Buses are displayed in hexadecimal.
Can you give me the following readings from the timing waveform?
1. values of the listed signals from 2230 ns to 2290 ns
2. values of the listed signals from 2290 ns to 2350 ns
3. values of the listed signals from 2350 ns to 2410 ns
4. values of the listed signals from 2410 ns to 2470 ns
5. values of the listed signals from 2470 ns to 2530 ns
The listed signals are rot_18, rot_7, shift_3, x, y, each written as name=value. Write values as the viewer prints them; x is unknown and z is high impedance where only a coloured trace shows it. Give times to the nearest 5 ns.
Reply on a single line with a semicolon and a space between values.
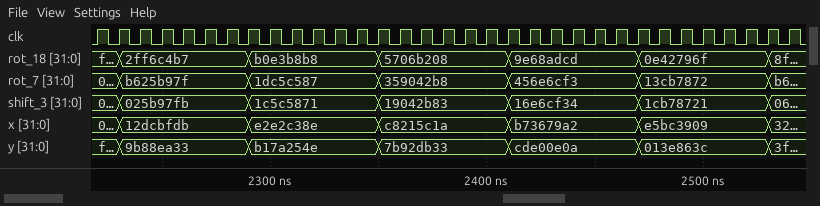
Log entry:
rot_18=2ff6c4b7, rot_7=b625b97f, shift_3=025b97fb, x=12dcbfdb, y=9b88ea33; rot_18=b0e3b8b8, rot_7=1dc5c587, shift_3=1c5c5871, x=e2e2c38e, y=b17a254e; rot_18=5706b208, rot_7=359042b8, shift_3=19042b83, x=c8215c1a, y=7b92db33; rot_18=9e68adcd, rot_7=456e6cf3, shift_3=16e6cf34, x=b73679a2, y=cde00e0a; rot_18=0e42796f, rot_7=13cb7872, shift_3=1cb78721, x=e5bc3909, y=013e863c
